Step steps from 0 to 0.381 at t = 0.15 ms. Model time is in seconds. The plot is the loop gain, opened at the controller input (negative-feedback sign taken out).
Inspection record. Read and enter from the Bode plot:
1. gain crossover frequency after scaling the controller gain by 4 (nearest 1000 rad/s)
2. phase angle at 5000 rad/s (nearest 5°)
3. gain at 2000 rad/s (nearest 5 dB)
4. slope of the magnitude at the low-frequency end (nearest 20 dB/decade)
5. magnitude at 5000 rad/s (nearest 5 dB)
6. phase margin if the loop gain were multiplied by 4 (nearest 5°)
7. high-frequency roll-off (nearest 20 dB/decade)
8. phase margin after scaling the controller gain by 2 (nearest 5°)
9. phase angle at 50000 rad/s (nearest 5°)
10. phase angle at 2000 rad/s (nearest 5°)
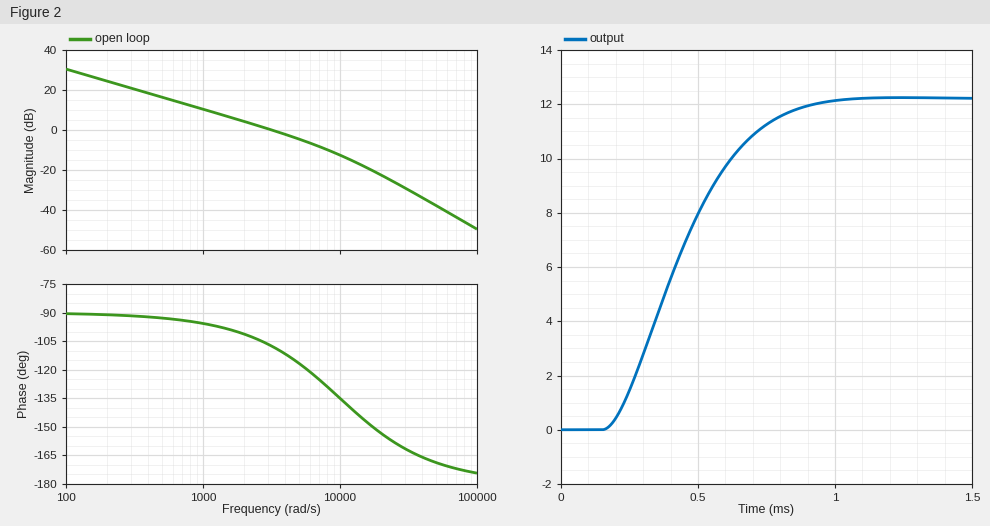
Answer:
10000 rad/s
-115°
5 dB
-20 dB/decade
-5 dB
45°
-40 dB/decade
60°
-170°
-100°
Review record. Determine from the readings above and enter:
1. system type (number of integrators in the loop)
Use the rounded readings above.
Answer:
1
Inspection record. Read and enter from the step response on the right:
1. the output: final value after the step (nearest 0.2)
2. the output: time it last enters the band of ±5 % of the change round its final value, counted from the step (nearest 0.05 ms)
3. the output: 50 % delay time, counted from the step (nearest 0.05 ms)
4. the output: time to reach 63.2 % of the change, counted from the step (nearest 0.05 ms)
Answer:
12.2
0.65 ms
0.25 ms
0.35 ms
